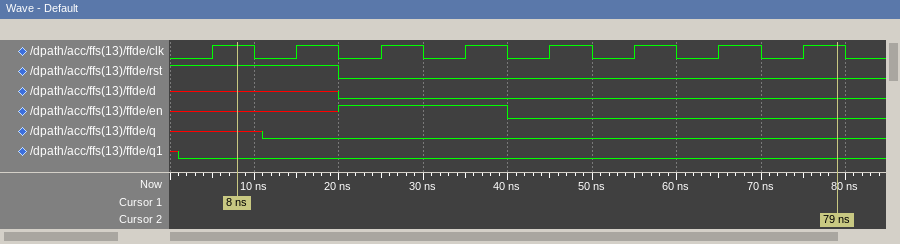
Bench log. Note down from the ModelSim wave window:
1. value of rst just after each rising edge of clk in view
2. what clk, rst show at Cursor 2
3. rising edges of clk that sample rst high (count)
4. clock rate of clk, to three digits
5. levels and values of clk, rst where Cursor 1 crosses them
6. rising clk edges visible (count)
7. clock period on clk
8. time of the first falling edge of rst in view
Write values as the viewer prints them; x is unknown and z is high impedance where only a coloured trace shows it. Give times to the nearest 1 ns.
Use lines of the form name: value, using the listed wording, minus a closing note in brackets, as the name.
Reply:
value of rst just after each rising edge of clk in view: 1 1 0 0 0 0 0 0
what clk, rst show at Cursor 2: clk=1, rst=0
rising edges of clk that sample rst high: 2
clock rate of clk, to three digits: 100 MHz
levels and values of clk, rst where Cursor 1 crosses them: clk=1, rst=1
rising clk edges visible: 8
clock period on clk: 10 ns
time of the first falling edge of rst in view: 20 ns
